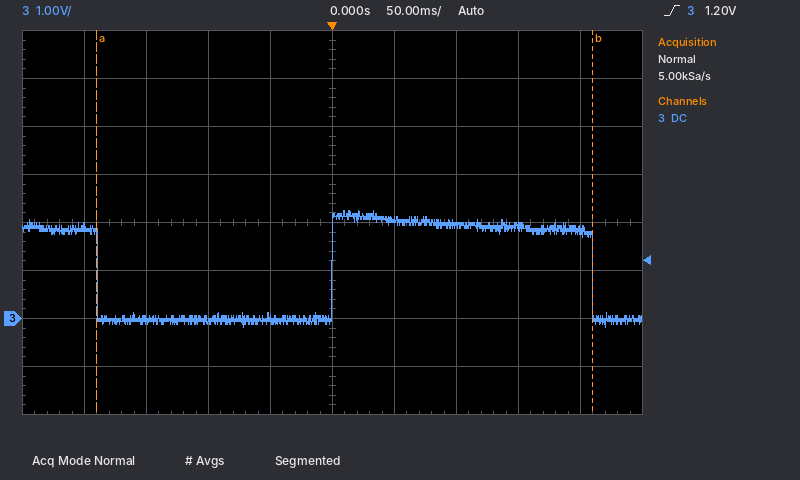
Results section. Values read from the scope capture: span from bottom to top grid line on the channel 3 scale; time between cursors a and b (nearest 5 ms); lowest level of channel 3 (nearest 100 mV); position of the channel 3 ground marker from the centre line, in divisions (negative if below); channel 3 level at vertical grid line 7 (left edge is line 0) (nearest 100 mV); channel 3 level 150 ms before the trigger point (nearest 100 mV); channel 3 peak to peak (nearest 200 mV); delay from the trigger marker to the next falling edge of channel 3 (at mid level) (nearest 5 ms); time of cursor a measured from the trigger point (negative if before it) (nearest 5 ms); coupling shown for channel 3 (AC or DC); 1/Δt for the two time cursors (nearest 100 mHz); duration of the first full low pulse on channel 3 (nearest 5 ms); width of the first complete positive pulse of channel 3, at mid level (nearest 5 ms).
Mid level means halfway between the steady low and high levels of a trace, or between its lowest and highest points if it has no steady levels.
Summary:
8 V
400 ms
-200 mV
-2.0 div
1.9 V
0.0 V
2.4 V
210 ms
-190 ms
DC
2.5 Hz
190 ms
210 ms
